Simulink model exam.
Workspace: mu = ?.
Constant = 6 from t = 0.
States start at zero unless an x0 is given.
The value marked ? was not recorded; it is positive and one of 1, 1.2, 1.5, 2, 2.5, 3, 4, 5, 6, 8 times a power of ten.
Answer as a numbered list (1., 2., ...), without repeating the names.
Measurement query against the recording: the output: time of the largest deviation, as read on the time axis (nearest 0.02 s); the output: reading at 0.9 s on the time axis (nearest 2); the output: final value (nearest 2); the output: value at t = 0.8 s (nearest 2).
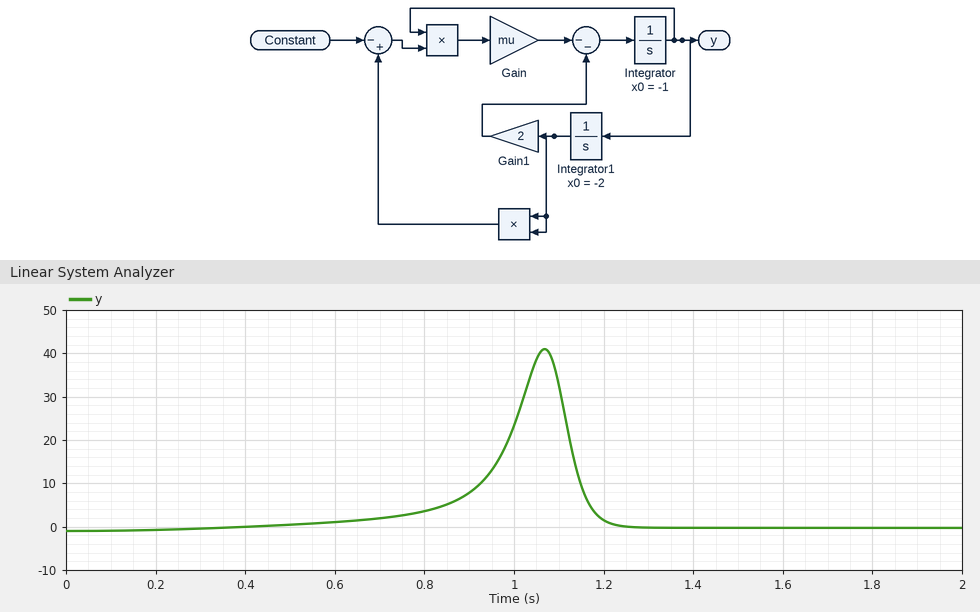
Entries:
1. 1.06 s
2. 8
3. 0
4. 4
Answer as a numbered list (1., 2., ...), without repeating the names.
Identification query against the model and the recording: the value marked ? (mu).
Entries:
1. 2
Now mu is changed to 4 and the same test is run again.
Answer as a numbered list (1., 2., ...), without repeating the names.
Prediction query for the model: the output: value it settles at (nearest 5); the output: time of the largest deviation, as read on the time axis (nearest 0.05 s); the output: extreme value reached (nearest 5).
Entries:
1. 0
2. 1.25 s
3. 80
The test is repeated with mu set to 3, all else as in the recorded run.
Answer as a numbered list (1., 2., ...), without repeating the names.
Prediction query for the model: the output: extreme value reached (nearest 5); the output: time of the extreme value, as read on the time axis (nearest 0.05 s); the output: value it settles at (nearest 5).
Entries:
1. 60
2. 1.15 s
3. 0
